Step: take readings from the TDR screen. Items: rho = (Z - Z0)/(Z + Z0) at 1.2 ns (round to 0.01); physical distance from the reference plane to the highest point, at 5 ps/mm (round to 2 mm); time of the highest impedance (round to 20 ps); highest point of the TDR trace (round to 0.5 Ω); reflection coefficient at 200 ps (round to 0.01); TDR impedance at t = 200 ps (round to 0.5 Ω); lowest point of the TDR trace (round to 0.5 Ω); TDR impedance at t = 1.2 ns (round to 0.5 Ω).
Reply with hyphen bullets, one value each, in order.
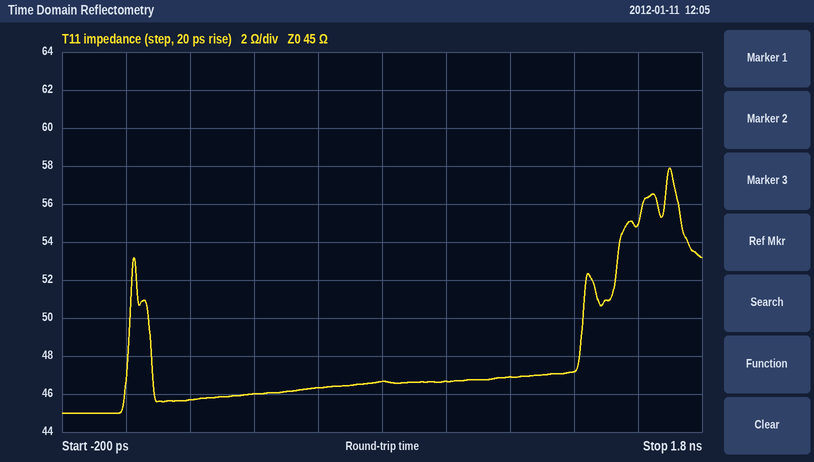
- +0.02
- 170 mm
- 1.70 ns
- 58.0 Ω
- +0.01
- 45.5 Ω
- 45.0 Ω
- 47.0 Ω
